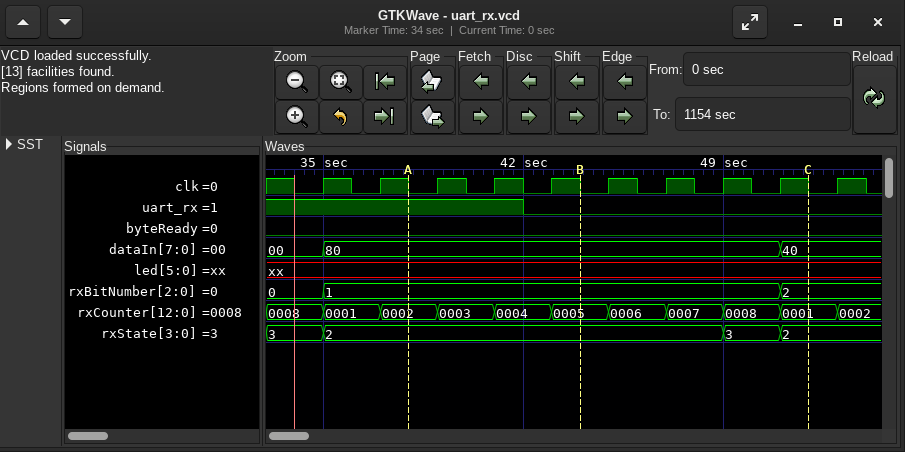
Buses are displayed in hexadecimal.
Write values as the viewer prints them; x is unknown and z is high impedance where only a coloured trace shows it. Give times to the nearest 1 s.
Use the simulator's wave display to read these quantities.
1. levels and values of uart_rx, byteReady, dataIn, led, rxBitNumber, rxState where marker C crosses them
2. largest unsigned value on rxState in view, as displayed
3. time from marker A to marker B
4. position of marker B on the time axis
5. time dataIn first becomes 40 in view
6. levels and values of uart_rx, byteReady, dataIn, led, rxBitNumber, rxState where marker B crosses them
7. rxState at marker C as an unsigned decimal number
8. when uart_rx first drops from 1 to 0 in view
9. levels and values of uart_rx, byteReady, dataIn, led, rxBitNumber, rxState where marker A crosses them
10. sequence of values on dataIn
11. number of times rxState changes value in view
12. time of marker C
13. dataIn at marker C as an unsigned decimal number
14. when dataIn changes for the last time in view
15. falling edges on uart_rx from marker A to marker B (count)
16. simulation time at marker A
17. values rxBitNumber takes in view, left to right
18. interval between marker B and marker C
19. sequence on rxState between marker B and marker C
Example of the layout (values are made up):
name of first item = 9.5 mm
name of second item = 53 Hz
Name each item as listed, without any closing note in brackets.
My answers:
levels and values of uart_rx, byteReady, dataIn, led, rxBitNumber, rxState where marker C crosses them = uart_rx=0, byteReady=0, dataIn=40, led=xx, rxBitNumber=2, rxState=2
largest unsigned value on rxState in view, as displayed = 3
time from marker A to marker B = 6 s
position of marker B on the time axis = 44 s
time dataIn first becomes 40 in view = 51 s
levels and values of uart_rx, byteReady, dataIn, led, rxBitNumber, rxState where marker B crosses them = uart_rx=0, byteReady=0, dataIn=80, led=xx, rxBitNumber=1, rxState=2
rxState at marker C as an unsigned decimal number = 2
when uart_rx first drops from 1 to 0 in view = 42 s
levels and values of uart_rx, byteReady, dataIn, led, rxBitNumber, rxState where marker A crosses them = uart_rx=1, byteReady=0, dataIn=80, led=xx, rxBitNumber=1, rxState=2
sequence of values on dataIn = 00, 80, 40
number of times rxState changes value in view = 3
time of marker C = 52 s
dataIn at marker C as an unsigned decimal number = 64
when dataIn changes for the last time in view = 51 s
falling edges on uart_rx from marker A to marker B = 1
simulation time at marker A = 38 s
values rxBitNumber takes in view, left to right = 0, 1, 2
interval between marker B and marker C = 8 s
sequence on rxState between marker B and marker C = 2, 3, 2
